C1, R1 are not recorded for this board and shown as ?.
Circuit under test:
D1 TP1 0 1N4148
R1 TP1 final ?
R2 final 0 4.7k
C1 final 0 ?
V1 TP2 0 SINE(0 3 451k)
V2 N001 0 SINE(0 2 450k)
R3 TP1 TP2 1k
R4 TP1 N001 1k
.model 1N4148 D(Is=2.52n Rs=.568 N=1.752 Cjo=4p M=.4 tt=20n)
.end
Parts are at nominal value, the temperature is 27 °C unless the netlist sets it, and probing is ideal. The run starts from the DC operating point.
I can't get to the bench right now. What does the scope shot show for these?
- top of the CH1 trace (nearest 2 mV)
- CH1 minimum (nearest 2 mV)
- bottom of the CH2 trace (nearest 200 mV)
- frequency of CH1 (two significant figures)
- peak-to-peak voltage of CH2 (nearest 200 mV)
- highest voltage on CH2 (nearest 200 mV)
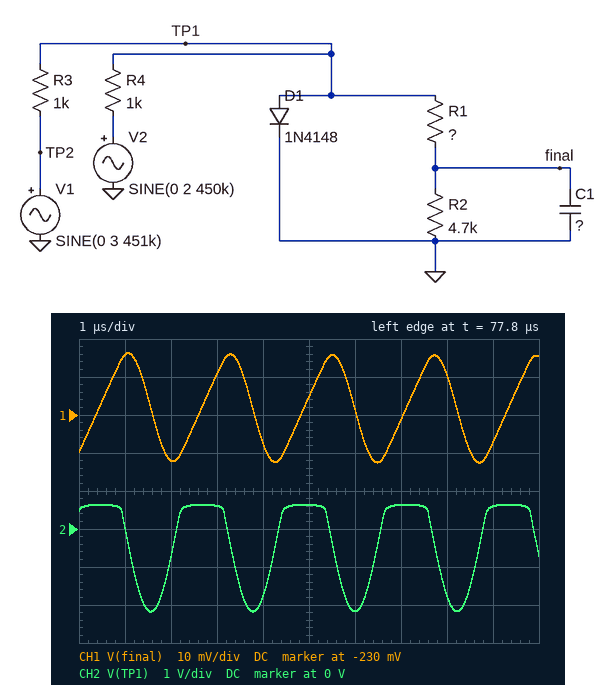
-214 mV
-242 mV
-2.2 V
450 kHz
2.8 V
600 mV
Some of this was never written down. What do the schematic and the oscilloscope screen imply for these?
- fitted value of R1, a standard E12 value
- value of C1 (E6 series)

3.9 kΩ
10 nF
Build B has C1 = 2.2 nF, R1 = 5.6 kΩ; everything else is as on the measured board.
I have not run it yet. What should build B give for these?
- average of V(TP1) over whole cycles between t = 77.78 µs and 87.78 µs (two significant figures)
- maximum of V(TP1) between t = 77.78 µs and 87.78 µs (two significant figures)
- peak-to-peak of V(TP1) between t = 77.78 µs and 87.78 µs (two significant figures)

-440 mV
640 mV
2.9 V
